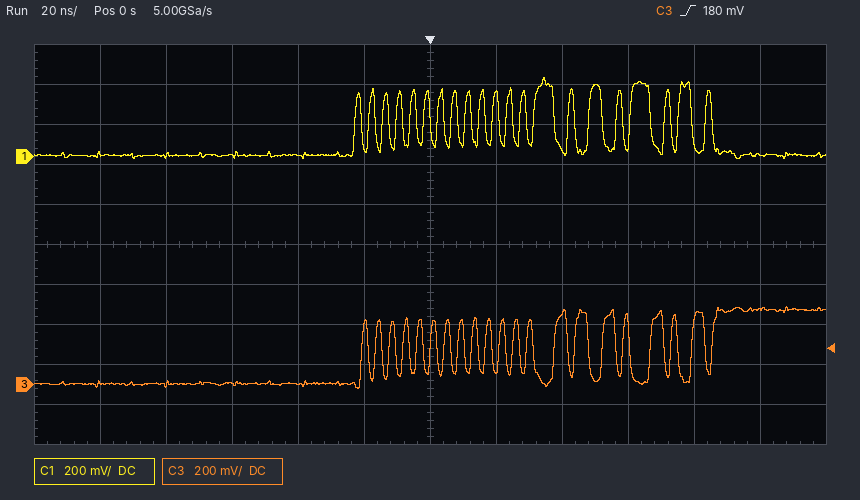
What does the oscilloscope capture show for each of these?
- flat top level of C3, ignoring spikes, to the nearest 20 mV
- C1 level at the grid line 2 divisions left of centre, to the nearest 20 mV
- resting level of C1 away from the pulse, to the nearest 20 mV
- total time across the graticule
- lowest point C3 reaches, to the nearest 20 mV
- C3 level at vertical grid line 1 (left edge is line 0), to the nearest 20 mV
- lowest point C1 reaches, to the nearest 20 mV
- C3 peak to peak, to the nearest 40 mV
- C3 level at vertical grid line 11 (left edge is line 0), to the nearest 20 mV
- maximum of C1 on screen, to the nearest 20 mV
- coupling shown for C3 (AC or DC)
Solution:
380 mV
0 mV
0 mV
240 ns
-20 mV
0 mV
-20 mV
400 mV
380 mV
400 mV
DC
